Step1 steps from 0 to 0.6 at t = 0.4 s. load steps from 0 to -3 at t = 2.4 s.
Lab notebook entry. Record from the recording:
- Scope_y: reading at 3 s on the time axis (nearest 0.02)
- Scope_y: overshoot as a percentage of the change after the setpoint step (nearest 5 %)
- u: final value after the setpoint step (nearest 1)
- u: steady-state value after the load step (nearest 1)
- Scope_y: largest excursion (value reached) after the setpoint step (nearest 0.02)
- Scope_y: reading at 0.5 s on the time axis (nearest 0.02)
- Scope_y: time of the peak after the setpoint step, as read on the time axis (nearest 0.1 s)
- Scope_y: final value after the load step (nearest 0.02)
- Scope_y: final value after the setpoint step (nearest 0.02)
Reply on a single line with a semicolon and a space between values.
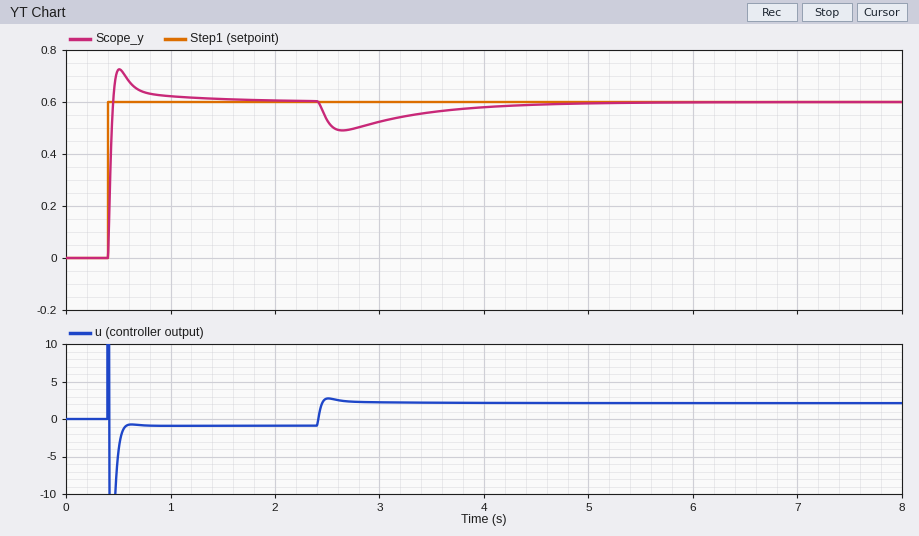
0.52; 20 %; -1; 2; 0.72; 0.72; 0.5 s; 0.60; 0.60
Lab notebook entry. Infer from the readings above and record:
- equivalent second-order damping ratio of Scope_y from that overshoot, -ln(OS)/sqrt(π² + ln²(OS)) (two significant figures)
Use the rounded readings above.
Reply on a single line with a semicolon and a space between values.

0.46
